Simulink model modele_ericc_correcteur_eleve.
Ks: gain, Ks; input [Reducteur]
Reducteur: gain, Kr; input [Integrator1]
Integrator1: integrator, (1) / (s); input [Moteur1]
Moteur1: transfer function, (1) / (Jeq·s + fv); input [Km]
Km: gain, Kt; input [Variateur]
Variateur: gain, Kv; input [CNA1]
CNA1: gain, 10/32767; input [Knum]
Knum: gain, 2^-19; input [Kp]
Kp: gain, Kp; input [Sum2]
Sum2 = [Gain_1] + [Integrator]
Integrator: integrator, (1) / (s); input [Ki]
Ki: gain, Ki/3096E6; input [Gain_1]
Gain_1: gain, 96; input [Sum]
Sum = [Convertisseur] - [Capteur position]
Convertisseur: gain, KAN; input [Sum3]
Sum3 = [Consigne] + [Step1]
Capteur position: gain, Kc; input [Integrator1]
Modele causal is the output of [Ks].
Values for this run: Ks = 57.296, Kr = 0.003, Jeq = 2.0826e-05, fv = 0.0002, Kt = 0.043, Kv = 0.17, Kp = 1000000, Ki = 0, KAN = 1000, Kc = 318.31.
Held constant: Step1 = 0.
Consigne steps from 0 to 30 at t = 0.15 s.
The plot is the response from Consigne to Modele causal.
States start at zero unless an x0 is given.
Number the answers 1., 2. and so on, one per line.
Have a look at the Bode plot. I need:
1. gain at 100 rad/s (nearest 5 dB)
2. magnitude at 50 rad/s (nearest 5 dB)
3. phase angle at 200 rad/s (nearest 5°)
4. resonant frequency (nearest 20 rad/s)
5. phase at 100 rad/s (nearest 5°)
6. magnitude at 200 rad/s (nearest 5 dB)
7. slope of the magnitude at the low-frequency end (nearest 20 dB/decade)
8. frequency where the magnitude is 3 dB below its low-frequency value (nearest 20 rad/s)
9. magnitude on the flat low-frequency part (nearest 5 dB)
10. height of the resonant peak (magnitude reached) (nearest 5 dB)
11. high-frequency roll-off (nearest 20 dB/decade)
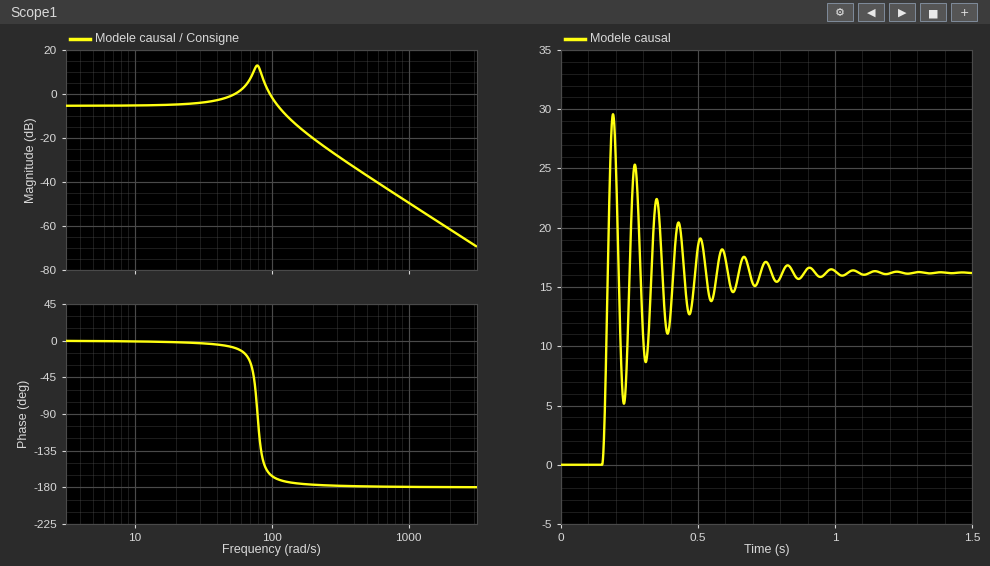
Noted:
1. 0 dB
2. 0 dB
3. -175°
4. 80 rad/s
5. -165°
6. -20 dB
7. 0 dB/decade
8. 120 rad/s
9. -5 dB
10. 15 dB
11. -40 dB/decade
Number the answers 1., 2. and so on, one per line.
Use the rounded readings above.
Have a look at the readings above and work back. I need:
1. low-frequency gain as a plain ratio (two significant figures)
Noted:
1. 0.56
